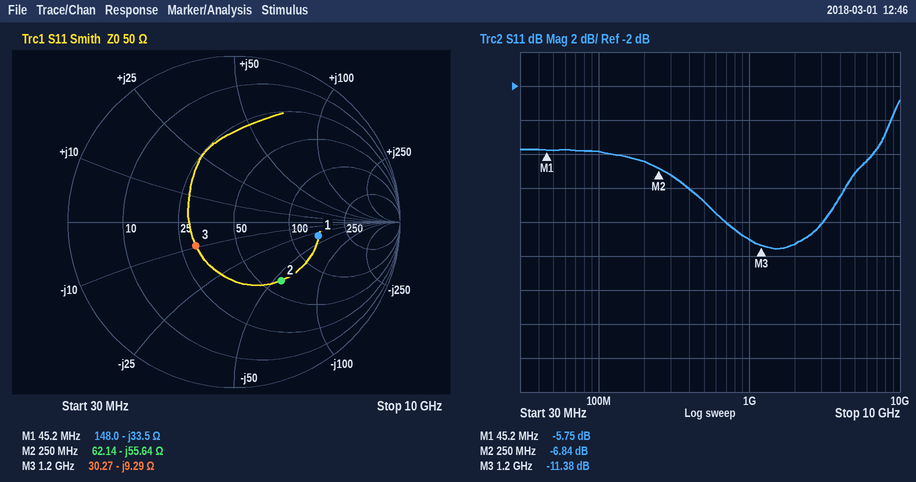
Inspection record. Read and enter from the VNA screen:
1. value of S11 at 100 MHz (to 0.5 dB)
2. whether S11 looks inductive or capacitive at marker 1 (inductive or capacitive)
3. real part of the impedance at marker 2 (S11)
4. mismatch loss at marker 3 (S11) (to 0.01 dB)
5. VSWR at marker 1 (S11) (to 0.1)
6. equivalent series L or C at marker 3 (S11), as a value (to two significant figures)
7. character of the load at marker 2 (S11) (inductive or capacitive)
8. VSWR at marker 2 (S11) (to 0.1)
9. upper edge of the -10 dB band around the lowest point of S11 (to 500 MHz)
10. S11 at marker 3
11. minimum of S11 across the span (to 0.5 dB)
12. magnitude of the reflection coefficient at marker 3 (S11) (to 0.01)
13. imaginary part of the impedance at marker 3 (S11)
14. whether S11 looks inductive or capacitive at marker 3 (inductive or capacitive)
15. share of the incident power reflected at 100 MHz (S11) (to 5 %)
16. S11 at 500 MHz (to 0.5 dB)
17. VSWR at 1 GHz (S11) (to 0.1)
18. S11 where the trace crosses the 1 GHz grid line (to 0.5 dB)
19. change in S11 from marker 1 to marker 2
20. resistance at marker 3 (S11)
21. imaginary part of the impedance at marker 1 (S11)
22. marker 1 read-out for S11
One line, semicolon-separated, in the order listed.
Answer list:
-6.0 dB; capacitive; 62.14 Ω; 0.33 dB; 3.1; 14 pF; capacitive; 2.7; 3.0 GHz; -11.38 dB; -11.5 dB; 0.27; -9.29 Ω; capacitive; 25 %; -9.0 dB; 1.8; -11.0 dB; -1.09 dB; 30.27 Ω; -33.5 Ω; -5.75 dB
